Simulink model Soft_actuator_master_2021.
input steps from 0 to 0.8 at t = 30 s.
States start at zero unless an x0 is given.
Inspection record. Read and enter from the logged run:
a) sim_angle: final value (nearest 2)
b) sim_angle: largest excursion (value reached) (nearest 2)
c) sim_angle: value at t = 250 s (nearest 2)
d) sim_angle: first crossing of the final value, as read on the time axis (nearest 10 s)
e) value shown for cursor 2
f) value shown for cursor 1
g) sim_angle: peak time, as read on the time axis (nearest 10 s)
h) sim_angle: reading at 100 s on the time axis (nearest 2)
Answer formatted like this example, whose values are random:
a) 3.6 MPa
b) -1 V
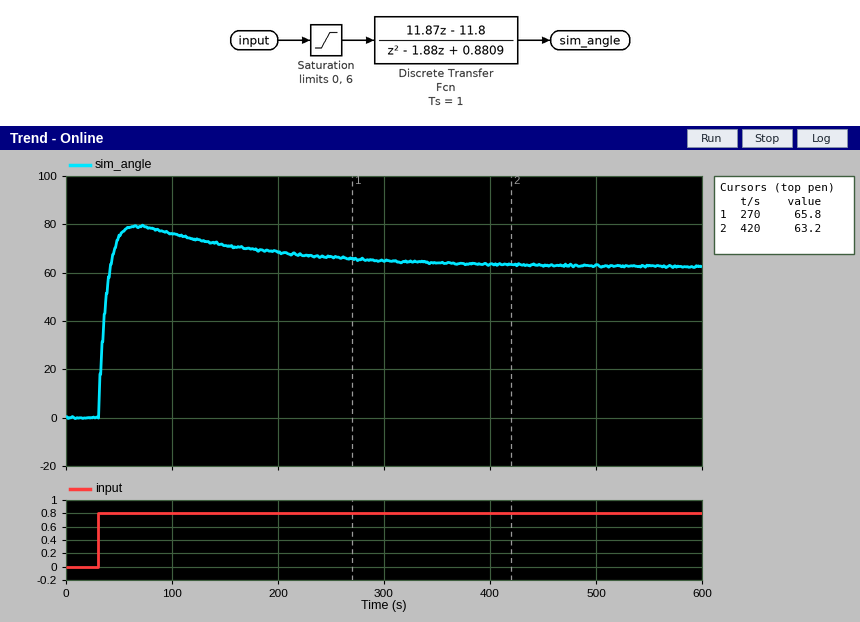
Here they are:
a) 62
b) 80
c) 66
d) 40 s
e) 63.2
f) 65.8
g) 70 s
h) 76
